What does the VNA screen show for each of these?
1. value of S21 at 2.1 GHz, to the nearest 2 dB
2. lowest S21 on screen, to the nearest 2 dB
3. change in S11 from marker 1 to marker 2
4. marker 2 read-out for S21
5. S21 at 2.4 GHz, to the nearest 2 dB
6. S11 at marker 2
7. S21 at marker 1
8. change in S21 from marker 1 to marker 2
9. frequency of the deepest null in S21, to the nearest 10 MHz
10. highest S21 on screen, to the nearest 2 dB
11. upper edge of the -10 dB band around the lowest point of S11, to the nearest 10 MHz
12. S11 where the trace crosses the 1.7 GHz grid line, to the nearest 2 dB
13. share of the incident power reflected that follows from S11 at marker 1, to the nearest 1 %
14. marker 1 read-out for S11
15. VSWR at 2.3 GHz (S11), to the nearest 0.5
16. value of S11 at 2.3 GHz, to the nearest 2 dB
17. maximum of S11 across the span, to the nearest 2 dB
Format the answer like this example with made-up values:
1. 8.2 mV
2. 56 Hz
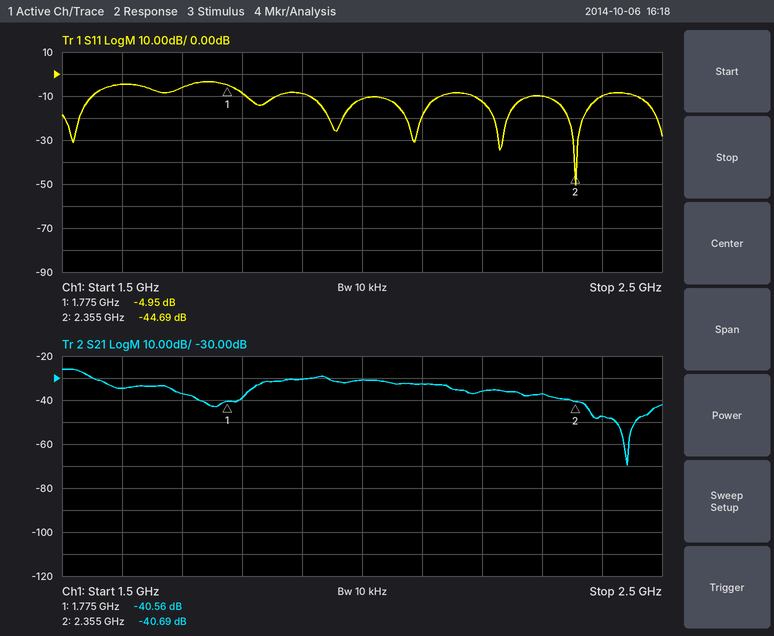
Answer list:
1. -32 dB
2. -70 dB
3. -39.74 dB
4. -40.69 dB
5. -48 dB
6. -44.69 dB
7. -40.56 dB
8. -0.13 dB
9. 2.44 GHz
10. -26 dB
11. 2.40 GHz
12. -6 dB
13. 32 %
14. -4.95 dB
15. 2.0
16. -10 dB
17. -4 dB
